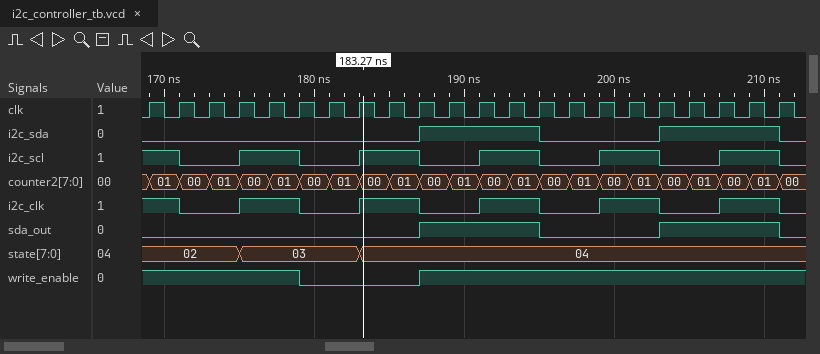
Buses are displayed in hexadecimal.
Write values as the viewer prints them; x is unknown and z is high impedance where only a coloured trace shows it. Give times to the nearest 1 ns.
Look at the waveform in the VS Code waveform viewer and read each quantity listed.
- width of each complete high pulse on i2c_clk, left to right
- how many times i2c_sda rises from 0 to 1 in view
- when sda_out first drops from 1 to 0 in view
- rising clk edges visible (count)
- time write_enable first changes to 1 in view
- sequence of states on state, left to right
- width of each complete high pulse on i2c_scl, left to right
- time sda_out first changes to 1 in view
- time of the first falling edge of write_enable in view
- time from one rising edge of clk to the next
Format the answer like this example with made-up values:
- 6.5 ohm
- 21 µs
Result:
- 4 ns, 4 ns, 4 ns, 4 ns, 4 ns
- 2
- 195 ns
- 22
- 187 ns
- 02, 03, 04
- 4 ns, 4 ns, 4 ns, 4 ns, 4 ns
- 187 ns
- 179 ns
- 2 ns
